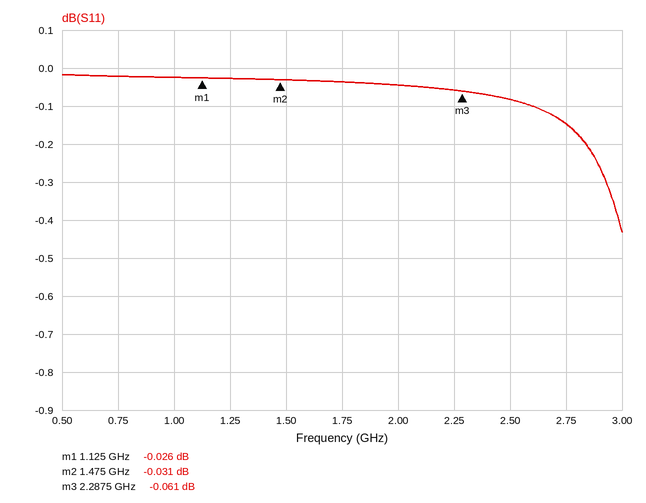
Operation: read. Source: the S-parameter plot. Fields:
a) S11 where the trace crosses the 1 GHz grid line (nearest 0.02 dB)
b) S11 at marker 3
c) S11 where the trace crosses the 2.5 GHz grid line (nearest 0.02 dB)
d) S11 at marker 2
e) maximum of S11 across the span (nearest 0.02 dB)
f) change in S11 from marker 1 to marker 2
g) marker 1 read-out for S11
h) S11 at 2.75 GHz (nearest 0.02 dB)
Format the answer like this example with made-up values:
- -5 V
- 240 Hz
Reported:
- -0.02 dB
- -0.061 dB
- -0.08 dB
- -0.031 dB
- -0.02 dB
- -0.005 dB
- -0.026 dB
- -0.14 dB
